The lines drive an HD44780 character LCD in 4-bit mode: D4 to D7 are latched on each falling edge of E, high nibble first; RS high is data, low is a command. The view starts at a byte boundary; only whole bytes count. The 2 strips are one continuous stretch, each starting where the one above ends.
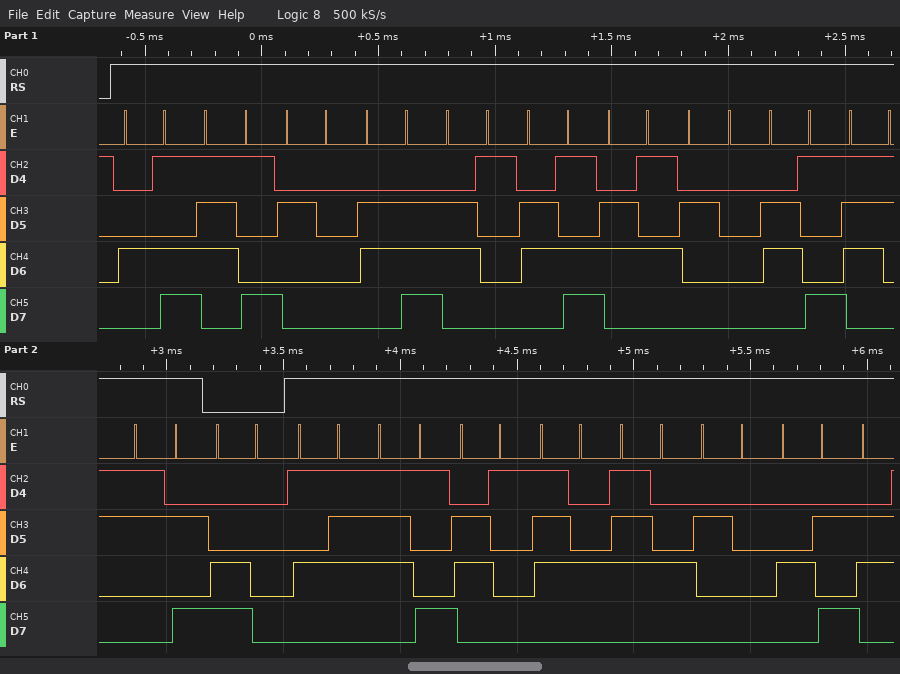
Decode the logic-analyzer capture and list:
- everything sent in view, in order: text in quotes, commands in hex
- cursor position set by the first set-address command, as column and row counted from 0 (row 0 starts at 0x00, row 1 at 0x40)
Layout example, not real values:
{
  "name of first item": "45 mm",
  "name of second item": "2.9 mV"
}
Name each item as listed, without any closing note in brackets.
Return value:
{
  "everything sent in view, in order: text in quotes, commands in hex": "\"My name is:\" 0xC0 \"Wyatt J\"",
  "cursor position set by the first set-address command, as column and row counted from 0": "column 0, row 1"
}
